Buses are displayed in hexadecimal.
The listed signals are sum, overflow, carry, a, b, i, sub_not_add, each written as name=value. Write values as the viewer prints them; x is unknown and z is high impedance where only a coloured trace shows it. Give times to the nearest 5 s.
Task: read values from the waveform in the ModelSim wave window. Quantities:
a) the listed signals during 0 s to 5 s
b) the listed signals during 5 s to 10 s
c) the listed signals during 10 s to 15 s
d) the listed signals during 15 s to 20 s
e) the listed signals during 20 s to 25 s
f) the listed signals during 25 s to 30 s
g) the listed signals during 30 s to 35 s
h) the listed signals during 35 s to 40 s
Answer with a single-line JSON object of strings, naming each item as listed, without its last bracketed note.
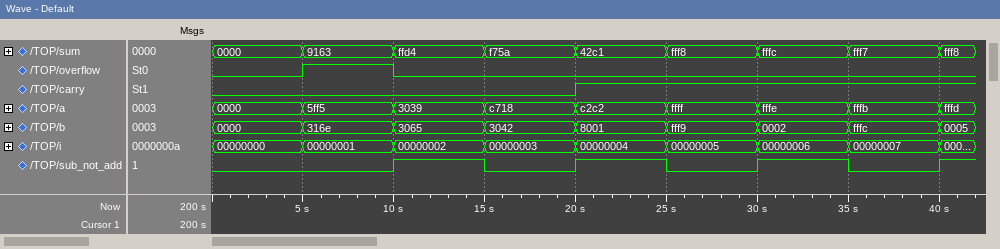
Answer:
{"the listed signals during 0 s to 5 s": "sum=0000, overflow=0, carry=0, a=0000, b=0000, i=00000000, sub_not_add=0", "the listed signals during 5 s to 10 s": "sum=9163, overflow=1, carry=0, a=5ff5, b=316e, i=00000001, sub_not_add=0", "the listed signals during 10 s to 15 s": "sum=ffd4, overflow=0, carry=0, a=3039, b=3065, i=00000002, sub_not_add=1", "the listed signals during 15 s to 20 s": "sum=f75a, overflow=0, carry=0, a=c718, b=3042, i=00000003, sub_not_add=0", "the listed signals during 20 s to 25 s": "sum=42c1, overflow=0, carry=1, a=c2c2, b=8001, i=00000004, sub_not_add=1", "the listed signals during 25 s to 30 s": "sum=fff8, overflow=0, carry=1, a=ffff, b=fff9, i=00000005, sub_not_add=0", "the listed signals during 30 s to 35 s": "sum=fffc, overflow=0, carry=1, a=fffe, b=0002, i=00000006, sub_not_add=1", "the listed signals during 35 s to 40 s": "sum=fff7, overflow=0, carry=1, a=fffb, b=fffc, i=00000007, sub_not_add=0"}
